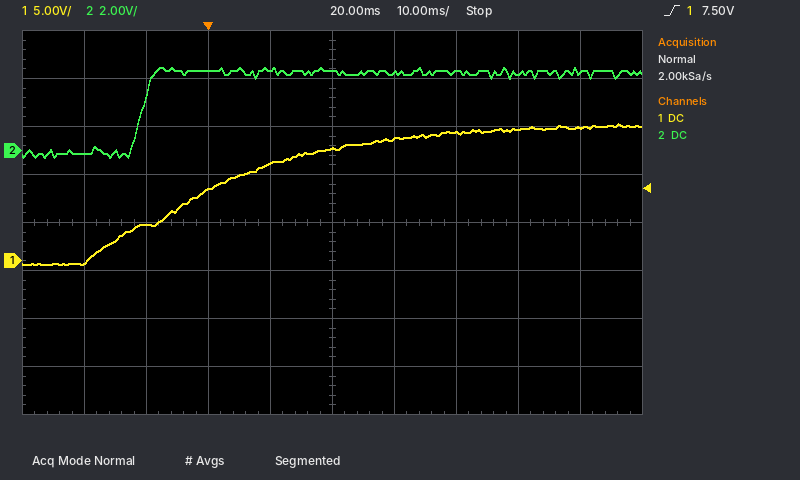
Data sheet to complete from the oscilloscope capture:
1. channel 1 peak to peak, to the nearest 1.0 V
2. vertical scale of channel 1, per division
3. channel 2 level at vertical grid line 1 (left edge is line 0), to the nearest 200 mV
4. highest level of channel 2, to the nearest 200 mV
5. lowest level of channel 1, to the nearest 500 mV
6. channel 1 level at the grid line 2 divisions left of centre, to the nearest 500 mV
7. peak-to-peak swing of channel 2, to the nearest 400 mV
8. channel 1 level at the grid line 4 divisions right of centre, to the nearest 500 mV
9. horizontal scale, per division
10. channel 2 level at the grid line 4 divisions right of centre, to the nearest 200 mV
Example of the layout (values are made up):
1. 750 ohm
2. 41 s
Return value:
1. 15.0 V
2. 5 V
3. -200 mV
4. 3.4 V
5. -500 mV
6. 7.5 V
7. 3.6 V
8. 14.0 V
9. 10 ms
10. 3.2 V
